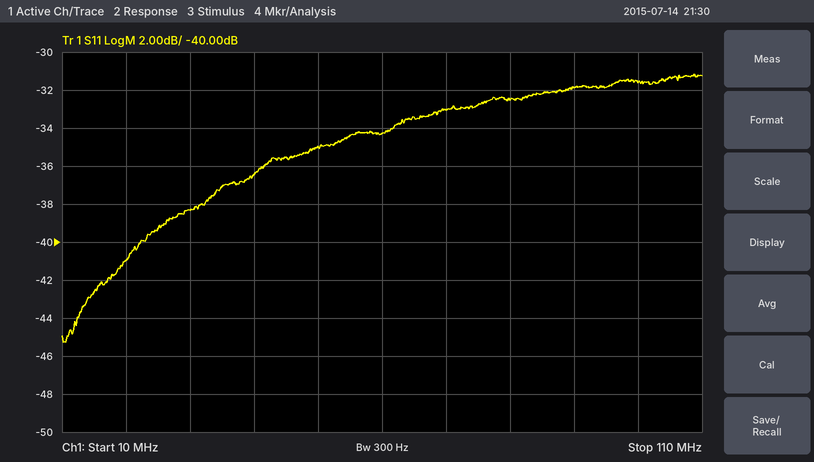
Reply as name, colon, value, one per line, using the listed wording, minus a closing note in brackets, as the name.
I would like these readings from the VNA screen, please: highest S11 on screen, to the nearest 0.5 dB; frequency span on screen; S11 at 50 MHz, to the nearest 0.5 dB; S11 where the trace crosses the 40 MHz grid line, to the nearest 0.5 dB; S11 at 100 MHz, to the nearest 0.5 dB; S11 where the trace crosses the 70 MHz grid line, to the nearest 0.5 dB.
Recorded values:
highest S11 on screen, to the nearest 0.5 dB: -31.0 dB
frequency span on screen: 100 MHz
S11 at 50 MHz, to the nearest 0.5 dB: -35.0 dB
S11 where the trace crosses the 40 MHz grid line, to the nearest 0.5 dB: -36.5 dB
S11 at 100 MHz, to the nearest 0.5 dB: -31.5 dB
S11 where the trace crosses the 70 MHz grid line, to the nearest 0.5 dB: -33.0 dB
